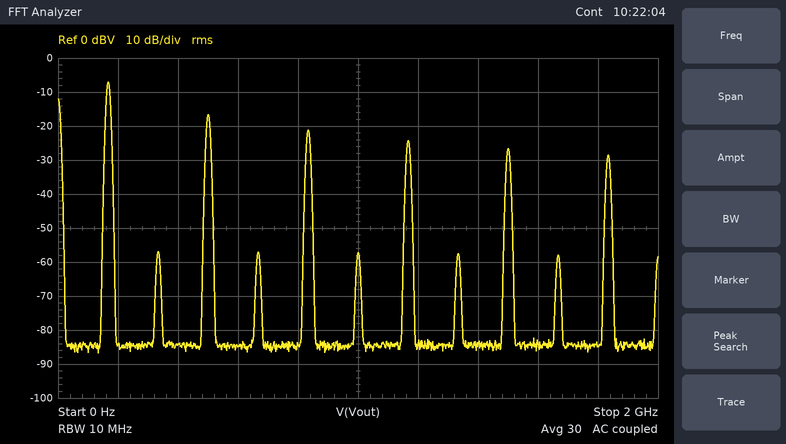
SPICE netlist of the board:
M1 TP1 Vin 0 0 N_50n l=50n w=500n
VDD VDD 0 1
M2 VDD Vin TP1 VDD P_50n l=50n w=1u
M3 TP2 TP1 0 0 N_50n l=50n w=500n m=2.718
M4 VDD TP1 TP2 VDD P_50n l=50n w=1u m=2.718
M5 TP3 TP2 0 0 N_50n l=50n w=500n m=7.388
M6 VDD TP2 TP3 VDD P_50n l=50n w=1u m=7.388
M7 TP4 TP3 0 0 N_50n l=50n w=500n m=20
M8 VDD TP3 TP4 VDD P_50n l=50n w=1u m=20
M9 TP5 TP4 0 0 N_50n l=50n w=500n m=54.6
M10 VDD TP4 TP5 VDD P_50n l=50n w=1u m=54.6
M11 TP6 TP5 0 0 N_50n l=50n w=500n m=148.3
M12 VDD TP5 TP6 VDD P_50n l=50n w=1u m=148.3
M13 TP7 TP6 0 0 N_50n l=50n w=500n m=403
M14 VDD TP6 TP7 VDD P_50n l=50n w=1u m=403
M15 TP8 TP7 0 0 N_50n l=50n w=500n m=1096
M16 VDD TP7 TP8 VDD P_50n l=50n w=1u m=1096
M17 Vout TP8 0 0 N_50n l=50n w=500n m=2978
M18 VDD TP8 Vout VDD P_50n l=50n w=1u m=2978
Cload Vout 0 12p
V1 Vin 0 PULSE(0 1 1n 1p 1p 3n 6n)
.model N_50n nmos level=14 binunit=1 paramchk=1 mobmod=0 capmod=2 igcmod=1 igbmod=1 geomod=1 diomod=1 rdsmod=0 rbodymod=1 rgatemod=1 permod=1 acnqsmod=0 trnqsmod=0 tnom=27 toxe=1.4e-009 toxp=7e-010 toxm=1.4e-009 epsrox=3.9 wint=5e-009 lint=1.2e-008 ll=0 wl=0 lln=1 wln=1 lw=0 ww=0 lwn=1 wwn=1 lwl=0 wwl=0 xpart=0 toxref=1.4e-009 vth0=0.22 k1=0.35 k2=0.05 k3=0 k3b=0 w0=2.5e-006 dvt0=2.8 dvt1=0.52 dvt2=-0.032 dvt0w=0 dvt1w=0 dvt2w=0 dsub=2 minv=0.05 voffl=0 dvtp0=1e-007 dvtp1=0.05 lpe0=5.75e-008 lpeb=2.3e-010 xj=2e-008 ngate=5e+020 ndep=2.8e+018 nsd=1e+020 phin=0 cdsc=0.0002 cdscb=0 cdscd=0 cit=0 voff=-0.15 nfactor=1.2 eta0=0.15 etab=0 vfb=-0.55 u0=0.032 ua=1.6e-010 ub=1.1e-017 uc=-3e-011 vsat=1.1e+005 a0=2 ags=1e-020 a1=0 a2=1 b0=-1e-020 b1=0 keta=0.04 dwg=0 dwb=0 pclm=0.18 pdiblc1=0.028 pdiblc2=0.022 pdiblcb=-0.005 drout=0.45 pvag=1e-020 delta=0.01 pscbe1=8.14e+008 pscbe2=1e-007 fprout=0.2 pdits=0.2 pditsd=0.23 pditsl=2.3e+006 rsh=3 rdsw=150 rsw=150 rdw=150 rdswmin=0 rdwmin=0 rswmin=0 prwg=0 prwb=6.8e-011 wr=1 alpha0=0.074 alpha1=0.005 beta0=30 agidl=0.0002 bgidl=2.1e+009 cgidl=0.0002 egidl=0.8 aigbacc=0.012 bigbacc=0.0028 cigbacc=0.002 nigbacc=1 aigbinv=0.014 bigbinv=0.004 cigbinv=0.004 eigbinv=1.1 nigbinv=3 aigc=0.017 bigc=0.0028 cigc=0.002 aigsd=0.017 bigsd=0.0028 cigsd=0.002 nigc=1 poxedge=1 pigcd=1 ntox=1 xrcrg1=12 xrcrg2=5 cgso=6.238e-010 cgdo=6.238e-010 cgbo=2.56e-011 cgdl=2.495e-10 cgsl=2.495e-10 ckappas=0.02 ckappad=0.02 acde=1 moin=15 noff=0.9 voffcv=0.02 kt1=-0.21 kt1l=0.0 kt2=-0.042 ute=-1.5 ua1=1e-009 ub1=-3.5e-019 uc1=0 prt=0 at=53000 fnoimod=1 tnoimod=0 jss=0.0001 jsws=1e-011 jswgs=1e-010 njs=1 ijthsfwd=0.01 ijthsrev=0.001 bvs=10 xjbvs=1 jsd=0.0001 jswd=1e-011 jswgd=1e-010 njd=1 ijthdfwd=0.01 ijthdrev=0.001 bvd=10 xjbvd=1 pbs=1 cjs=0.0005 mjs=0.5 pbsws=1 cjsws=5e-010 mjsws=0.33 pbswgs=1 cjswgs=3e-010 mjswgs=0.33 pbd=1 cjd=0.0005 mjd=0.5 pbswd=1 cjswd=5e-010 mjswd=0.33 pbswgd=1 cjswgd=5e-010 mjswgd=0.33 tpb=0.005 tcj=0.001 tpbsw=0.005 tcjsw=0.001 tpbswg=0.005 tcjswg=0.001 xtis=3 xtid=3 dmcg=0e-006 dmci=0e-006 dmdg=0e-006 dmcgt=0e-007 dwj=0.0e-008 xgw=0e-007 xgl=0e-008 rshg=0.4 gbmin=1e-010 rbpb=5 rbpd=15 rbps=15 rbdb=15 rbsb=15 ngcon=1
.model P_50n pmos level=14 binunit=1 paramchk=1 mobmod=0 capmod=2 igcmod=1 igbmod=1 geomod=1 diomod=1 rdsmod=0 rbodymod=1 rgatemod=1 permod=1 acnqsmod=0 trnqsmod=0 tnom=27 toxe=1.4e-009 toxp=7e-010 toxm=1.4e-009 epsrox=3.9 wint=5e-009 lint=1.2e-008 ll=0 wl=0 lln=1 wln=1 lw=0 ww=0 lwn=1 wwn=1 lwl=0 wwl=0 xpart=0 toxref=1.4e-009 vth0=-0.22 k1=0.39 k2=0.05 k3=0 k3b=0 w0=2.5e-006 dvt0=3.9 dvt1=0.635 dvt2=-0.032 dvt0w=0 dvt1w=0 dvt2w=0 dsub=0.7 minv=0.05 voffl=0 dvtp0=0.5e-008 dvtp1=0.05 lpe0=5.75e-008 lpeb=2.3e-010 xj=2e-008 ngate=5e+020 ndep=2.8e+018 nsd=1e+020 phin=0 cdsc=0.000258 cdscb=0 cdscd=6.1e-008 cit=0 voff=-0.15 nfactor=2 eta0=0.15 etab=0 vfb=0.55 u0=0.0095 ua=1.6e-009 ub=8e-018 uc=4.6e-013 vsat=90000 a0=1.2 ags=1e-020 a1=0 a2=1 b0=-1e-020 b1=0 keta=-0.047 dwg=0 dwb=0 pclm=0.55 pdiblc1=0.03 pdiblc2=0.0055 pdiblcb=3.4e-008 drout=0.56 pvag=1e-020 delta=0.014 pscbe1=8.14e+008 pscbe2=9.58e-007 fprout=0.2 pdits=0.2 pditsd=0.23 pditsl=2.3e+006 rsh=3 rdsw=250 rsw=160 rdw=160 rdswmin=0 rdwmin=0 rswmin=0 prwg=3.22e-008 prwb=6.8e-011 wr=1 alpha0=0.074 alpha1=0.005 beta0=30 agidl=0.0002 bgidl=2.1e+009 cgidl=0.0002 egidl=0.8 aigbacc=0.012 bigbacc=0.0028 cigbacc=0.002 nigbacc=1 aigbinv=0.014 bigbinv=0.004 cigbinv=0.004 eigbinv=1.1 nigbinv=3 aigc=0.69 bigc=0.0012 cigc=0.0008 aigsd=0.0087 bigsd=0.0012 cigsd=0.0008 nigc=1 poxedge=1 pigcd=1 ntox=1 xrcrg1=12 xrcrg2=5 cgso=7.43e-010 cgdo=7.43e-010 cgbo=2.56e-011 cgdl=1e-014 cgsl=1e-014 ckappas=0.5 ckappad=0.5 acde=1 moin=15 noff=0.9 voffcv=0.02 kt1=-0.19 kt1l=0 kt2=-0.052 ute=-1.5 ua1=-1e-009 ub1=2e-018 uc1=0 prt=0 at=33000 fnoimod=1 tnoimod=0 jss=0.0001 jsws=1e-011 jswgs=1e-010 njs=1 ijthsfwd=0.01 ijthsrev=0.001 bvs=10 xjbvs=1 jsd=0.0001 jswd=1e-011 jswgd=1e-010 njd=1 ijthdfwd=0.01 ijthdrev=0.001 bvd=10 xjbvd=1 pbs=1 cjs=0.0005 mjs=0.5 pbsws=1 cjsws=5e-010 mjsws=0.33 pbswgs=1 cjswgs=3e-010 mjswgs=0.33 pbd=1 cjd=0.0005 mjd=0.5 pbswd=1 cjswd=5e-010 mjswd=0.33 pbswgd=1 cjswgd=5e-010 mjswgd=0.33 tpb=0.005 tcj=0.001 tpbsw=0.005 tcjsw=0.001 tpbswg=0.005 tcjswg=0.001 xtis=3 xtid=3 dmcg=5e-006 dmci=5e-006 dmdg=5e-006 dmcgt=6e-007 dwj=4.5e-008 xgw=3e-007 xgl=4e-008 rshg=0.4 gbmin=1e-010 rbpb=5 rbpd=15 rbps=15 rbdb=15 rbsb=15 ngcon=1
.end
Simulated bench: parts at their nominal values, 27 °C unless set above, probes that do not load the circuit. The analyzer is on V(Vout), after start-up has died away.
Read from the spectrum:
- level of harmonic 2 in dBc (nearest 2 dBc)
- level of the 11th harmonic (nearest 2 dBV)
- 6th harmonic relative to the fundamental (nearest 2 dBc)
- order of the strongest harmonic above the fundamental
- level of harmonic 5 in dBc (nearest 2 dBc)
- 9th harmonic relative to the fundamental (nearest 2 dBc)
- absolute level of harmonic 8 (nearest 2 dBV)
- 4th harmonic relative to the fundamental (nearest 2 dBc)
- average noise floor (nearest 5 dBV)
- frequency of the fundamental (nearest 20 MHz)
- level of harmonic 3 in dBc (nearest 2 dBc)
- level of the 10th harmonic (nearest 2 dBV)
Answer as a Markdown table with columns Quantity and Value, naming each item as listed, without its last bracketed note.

| Quantity | Value |
|---|---|
| level of harmonic 2 in dBc | -50 dBc |
| level of the 11th harmonic | -28 dBV |
| 6th harmonic relative to the fundamental | -50 dBc |
| order of the strongest harmonic above the fundamental | 3 |
| level of harmonic 5 in dBc | -14 dBc |
| 9th harmonic relative to the fundamental | -20 dBc |
| absolute level of harmonic 8 | -58 dBV |
| 4th harmonic relative to the fundamental | -50 dBc |
| average noise floor | -85 dBV |
| frequency of the fundamental | 160 MHz |
| level of harmonic 3 in dBc | -10 dBc |
| level of the 10th harmonic | -58 dBV |
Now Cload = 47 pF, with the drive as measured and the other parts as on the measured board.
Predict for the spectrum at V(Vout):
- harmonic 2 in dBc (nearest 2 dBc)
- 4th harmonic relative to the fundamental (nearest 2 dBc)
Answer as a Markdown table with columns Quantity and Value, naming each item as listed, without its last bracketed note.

| Quantity | Value |
|---|---|
| harmonic 2 in dBc | -48 dBc |
| 4th harmonic relative to the fundamental | -48 dBc |
